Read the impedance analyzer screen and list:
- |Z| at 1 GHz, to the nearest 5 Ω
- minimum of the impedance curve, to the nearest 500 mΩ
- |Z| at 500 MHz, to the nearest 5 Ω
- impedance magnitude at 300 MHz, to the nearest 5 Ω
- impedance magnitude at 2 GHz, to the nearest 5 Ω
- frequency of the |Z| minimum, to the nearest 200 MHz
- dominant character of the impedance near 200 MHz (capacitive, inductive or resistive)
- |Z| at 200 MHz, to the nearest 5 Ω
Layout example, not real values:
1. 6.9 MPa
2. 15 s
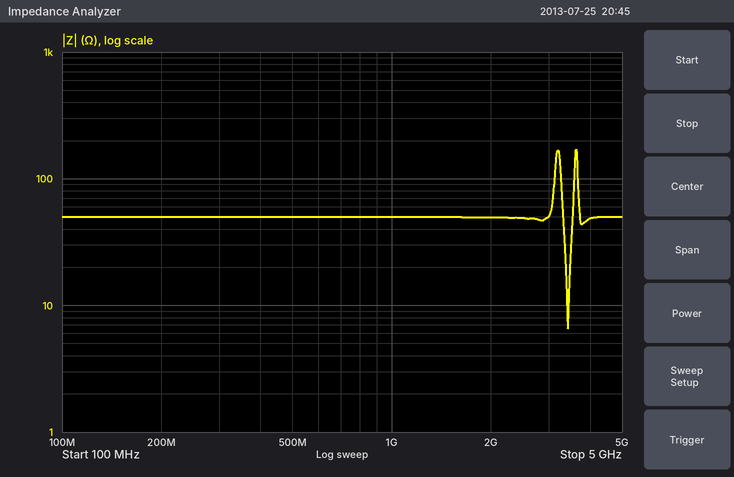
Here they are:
1. 50 Ω
2. 6.5 Ω
3. 50 Ω
4. 50 Ω
5. 50 Ω
6. 3.4 GHz
7. resistive
8. 50 Ω
